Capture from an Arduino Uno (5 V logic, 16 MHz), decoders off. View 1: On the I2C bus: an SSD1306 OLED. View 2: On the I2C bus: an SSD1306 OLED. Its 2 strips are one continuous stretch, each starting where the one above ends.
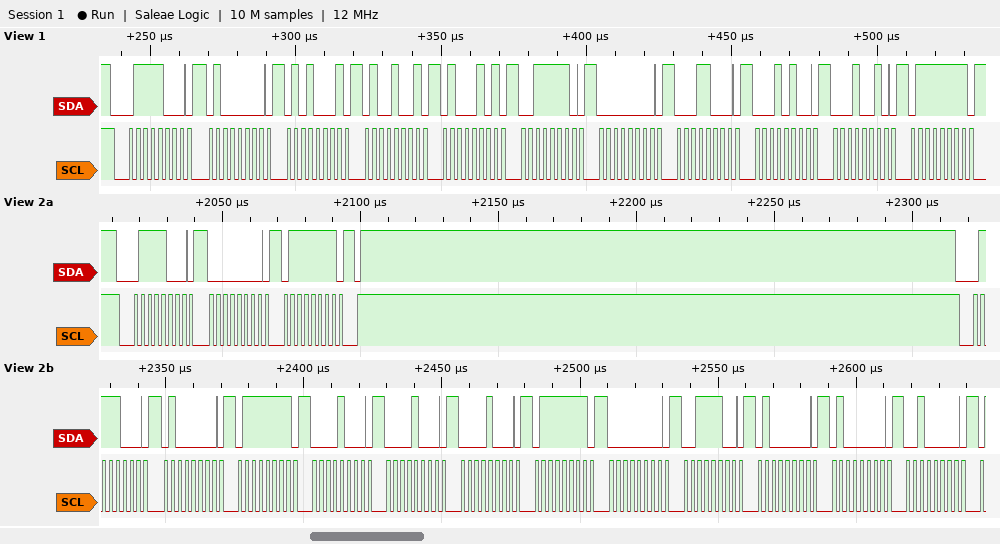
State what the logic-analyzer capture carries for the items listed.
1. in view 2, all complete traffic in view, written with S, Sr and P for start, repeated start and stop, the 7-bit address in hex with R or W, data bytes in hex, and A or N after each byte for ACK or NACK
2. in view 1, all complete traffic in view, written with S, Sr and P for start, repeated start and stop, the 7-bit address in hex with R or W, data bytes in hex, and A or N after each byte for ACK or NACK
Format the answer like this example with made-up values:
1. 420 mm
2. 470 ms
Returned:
1. S 3CW A 00 A 7F A P S 3CW A 40 A 7F A 08 A 08 A 08 A 7F A 00 A 3C A 40 A 40 A 20 A
2. S 3CW A 40 A 51 A 49 A 45 A 3E A 00 A 18 A 14 A 12 A 7F A
